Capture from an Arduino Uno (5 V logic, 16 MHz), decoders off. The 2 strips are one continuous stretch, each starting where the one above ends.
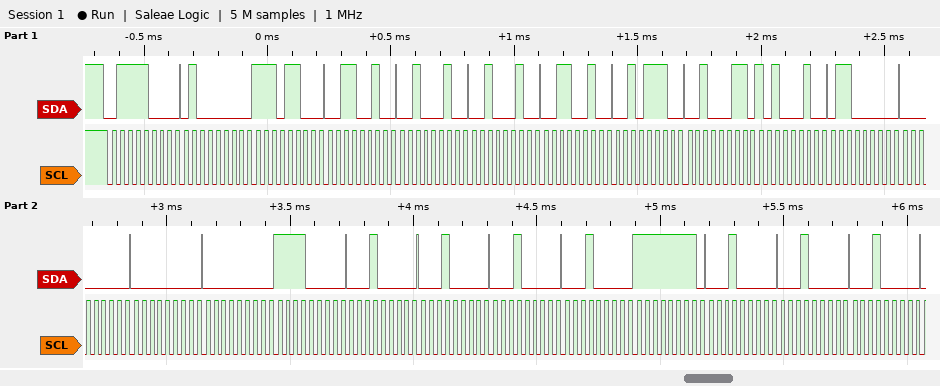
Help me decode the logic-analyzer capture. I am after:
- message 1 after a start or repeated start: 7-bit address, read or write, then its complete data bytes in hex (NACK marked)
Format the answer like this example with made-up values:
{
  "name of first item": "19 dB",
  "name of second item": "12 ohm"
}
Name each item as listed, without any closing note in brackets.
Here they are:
{
  "message 1 after a start or repeated start: 7-bit address, read or write, then its complete data bytes in hex": "0x3C write: 40 EC 32 22 22 32 2E 23 A2 60 00 00 00 F0 10 10 10 10 FF 10 10 10"
}
